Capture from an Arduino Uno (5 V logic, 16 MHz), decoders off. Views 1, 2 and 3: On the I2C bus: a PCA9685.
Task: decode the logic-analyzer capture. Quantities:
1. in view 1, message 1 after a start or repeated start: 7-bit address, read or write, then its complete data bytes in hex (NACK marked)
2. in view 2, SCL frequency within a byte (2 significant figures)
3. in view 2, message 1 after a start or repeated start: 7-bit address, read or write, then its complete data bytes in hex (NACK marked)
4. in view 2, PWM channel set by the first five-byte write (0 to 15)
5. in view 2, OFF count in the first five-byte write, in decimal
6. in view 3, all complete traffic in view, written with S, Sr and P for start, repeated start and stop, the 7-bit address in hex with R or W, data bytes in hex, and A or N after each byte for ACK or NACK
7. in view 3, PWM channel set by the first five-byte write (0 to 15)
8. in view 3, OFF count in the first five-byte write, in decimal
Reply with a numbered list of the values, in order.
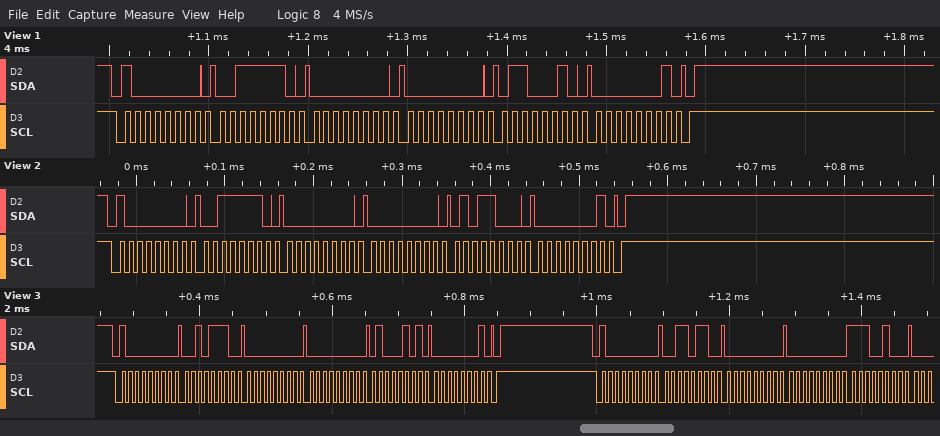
1. 0x40 write: 3E 00 00 62 01
2. 100 kHz
3. 0x40 write: 3E 00 00 58 01
4. 14
5. 344
6. S 40W A 2E A 00 A 00 A 45 A 01 A P S 40W A 36 A 00 A 00 A E4 A
7. 10
8. 325
